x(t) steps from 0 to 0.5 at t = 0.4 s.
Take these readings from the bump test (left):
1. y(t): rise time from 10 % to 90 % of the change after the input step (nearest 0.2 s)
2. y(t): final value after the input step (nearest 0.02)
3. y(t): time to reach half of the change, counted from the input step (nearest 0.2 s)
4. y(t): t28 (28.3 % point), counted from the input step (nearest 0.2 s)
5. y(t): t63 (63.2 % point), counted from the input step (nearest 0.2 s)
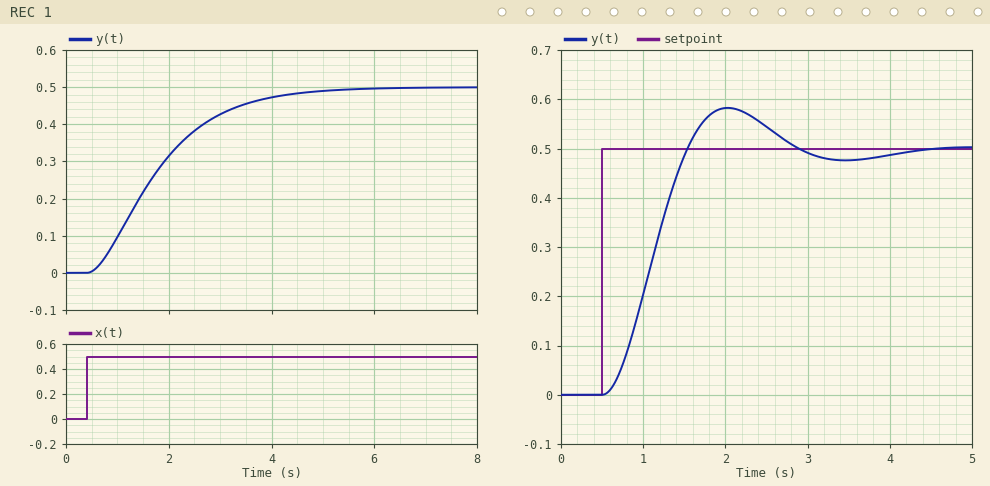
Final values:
2.6 s
0.50
1.2 s
0.8 s
1.6 s
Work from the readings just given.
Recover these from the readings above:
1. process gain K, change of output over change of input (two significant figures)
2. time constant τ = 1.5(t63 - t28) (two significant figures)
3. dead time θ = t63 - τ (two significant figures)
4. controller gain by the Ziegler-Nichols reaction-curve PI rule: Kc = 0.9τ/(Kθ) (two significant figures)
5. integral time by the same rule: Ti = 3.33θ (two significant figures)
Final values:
1.0
1.2 s
0.40 s
2.7
1.3 s
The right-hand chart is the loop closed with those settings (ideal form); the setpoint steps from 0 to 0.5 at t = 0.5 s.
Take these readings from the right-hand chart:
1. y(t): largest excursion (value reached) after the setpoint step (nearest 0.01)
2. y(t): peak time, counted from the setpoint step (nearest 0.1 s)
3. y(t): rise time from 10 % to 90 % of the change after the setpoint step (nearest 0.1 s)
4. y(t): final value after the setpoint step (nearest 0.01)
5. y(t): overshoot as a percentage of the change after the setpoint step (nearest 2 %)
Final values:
0.58
1.5 s
0.7 s
0.50
16 %
